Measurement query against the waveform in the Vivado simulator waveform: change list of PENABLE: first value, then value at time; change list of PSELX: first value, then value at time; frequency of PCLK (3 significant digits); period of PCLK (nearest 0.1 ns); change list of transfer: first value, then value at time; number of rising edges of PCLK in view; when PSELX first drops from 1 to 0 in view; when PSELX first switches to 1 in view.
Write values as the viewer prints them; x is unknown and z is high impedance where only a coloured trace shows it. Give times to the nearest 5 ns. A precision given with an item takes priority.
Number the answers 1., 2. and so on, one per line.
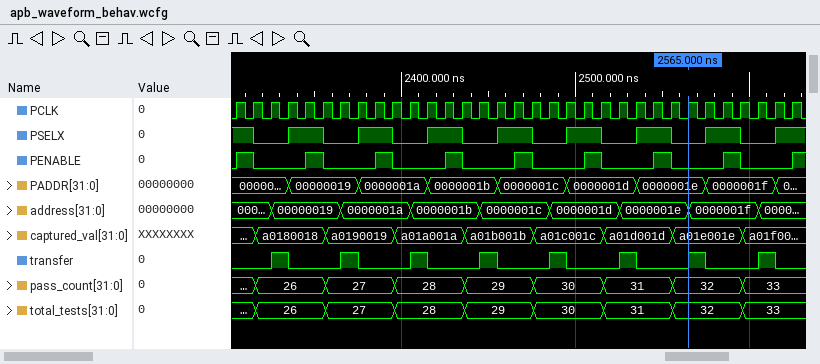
1. 0, 1 at 2305 ns, 0 at 2315 ns, 1 at 2345 ns, 0 at 2355 ns, 1 at 2385 ns, 0 at 2395 ns, 1 at 2425 ns, 0 at 2435 ns, 1 at 2465 ns, 0 at 2475 ns, 1 at 2505 ns, 0 at 2515 ns, 1 at 2545 ns, 0 at 2555 ns, 1 at 2585 ns, 0 at 2595 ns, 1 at 2625 ns
2. 1, 0 at 2315 ns, 1 at 2335 ns, 0 at 2355 ns, 1 at 2375 ns, 0 at 2395 ns, 1 at 2415 ns, 0 at 2435 ns, 1 at 2455 ns, 0 at 2475 ns, 1 at 2495 ns, 0 at 2515 ns, 1 at 2535 ns, 0 at 2555 ns, 1 at 2575 ns, 0 at 2595 ns, 1 at 2615 ns
3. 100 MHz
4. 10 ns
5. 0, 1 at 2325 ns, 0 at 2335 ns, 1 at 2365 ns, 0 at 2375 ns, 1 at 2405 ns, 0 at 2415 ns, 1 at 2445 ns, 0 at 2455 ns, 1 at 2485 ns, 0 at 2495 ns, 1 at 2525 ns, 0 at 2535 ns, 1 at 2565 ns, 0 at 2575 ns, 1 at 2605 ns, 0 at 2615 ns
6. 33
7. 2315 ns
8. 2335 ns
